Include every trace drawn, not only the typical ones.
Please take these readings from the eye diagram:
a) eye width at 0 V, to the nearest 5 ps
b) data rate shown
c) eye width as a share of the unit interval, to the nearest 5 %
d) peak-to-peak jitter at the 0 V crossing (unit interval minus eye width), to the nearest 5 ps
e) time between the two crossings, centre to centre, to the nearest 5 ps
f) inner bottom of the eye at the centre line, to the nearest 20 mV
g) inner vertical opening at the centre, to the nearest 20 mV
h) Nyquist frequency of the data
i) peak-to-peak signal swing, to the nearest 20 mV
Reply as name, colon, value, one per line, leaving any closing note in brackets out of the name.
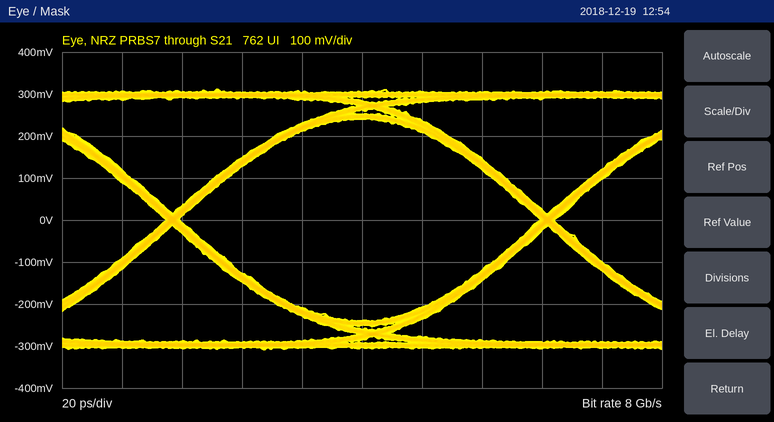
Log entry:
eye width at 0 V, to the nearest 5 ps: 120 ps
data rate shown: 8 Gb/s
eye width as a share of the unit interval, to the nearest 5 %: 95 %
peak-to-peak jitter at the 0 V crossing (unit interval minus eye width), to the nearest 5 ps: 5 ps
time between the two crossings, centre to centre, to the nearest 5 ps: 125 ps
inner bottom of the eye at the centre line, to the nearest 20 mV: -240 mV
inner vertical opening at the centre, to the nearest 20 mV: 480 mV
Nyquist frequency of the data: 4 GHz
peak-to-peak signal swing, to the nearest 20 mV: 620 mV
